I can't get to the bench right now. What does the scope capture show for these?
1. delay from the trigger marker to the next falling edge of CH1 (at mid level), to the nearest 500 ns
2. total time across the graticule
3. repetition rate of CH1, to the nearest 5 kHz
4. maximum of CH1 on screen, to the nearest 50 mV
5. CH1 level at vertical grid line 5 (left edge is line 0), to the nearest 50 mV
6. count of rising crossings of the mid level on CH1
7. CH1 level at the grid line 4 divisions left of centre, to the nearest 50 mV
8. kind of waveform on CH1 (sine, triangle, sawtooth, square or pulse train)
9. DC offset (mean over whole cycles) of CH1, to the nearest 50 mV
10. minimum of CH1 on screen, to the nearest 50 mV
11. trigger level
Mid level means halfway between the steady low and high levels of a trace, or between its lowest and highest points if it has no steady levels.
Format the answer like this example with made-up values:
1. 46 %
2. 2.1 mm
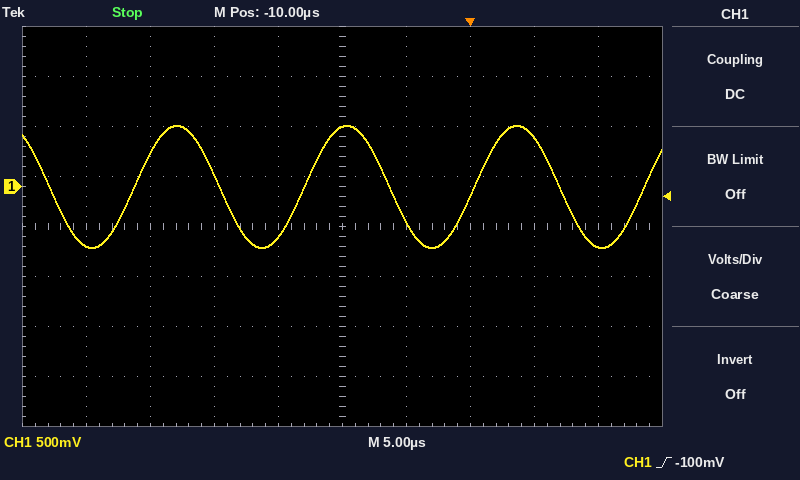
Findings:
1. 7.0 µs
2. 50 µs
3. 75 kHz
4. 600 mV
5. 600 mV
6. 4
7. -600 mV
8. sine
9. 0 mV
10. -600 mV
11. -100 mV
